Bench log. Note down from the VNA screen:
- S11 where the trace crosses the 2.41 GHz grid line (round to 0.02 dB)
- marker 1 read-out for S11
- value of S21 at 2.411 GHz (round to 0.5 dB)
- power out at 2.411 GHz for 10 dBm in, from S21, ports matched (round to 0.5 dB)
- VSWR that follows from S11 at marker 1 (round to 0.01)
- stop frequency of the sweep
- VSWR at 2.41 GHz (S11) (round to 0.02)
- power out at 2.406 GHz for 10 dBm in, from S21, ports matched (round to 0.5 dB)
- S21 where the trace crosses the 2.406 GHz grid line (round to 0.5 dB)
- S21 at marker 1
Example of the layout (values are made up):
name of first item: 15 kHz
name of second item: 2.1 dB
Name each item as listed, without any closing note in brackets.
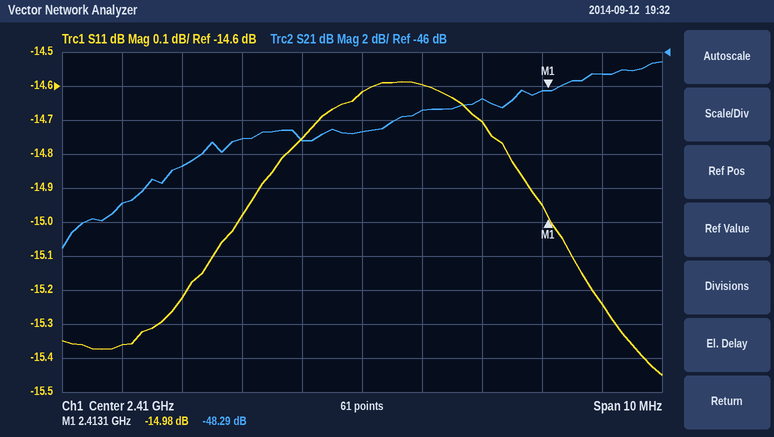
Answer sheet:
S11 where the trace crosses the 2.41 GHz grid line: -14.62 dB
marker 1 read-out for S11: -14.98 dB
value of S21 at 2.411 GHz: -49.5 dB
power out at 2.411 GHz for 10 dBm in, from S21, ports matched: -39.5 dBm
VSWR that follows from S11 at marker 1: 1.43
stop frequency of the sweep: 2.415 GHz
VSWR at 2.41 GHz (S11): 1.46
power out at 2.406 GHz for 10 dBm in, from S21, ports matched: -45.0 dBm
S21 where the trace crosses the 2.406 GHz grid line: -55.0 dB
S21 at marker 1: -48.29 dB
